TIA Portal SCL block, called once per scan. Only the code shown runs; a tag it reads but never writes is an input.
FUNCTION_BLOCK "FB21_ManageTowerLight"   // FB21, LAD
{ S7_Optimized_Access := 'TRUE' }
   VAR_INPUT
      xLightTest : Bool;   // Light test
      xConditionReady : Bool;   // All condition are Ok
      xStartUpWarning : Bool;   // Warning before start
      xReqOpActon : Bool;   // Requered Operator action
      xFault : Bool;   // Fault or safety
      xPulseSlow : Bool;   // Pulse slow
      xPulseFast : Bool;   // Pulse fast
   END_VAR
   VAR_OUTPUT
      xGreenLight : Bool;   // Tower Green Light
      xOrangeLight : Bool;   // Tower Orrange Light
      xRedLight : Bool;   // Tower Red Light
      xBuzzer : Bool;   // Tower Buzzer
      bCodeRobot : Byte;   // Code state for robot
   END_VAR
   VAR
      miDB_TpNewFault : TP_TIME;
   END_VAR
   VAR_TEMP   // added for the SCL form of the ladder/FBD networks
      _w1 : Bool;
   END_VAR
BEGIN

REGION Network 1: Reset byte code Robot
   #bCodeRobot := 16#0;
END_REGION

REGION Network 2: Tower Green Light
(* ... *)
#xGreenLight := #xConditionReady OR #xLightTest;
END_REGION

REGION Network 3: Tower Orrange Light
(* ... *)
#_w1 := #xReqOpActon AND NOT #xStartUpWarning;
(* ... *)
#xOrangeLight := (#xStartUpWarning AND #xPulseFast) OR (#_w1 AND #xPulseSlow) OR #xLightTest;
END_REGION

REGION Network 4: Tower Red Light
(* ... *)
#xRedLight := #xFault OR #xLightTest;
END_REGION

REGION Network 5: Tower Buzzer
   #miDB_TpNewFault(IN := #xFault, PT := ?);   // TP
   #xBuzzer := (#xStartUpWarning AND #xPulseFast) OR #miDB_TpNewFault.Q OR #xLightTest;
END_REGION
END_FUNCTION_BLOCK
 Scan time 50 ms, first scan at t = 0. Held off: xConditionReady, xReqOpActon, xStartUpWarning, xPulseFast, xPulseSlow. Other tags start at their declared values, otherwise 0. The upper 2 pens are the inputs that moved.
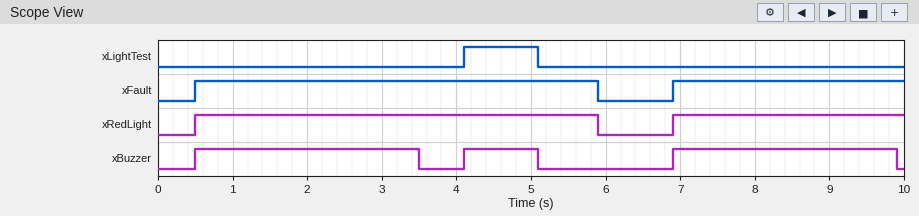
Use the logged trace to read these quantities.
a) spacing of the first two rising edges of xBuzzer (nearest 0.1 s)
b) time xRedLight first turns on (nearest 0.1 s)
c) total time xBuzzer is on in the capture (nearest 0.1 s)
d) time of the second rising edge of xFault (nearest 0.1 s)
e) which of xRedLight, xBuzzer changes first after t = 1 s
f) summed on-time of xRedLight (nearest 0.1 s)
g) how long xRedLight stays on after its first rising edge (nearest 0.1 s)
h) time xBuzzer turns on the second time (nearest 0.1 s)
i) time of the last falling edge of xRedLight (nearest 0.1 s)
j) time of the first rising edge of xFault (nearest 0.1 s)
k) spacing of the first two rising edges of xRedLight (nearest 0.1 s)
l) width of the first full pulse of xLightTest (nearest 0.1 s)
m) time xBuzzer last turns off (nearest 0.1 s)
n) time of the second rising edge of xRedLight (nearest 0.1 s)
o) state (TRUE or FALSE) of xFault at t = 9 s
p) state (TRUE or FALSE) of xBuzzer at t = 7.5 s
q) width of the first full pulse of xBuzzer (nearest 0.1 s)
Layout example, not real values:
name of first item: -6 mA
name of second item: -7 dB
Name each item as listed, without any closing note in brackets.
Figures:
spacing of the first two rising edges of xBuzzer: 3.6 s
time xRedLight first turns on: 0.5 s
total time xBuzzer is on in the capture: 7.0 s
time of the second rising edge of xFault: 6.9 s
which of xRedLight, xBuzzer changes first after t = 1 s: xBuzzer
summed on-time of xRedLight: 8.5 s
how long xRedLight stays on after its first rising edge: 5.4 s
time xBuzzer turns on the second time: 4.1 s
time of the last falling edge of xRedLight: 5.9 s
time of the first rising edge of xFault: 0.5 s
spacing of the first two rising edges of xRedLight: 6.4 s
width of the first full pulse of xLightTest: 1.0 s
time xBuzzer last turns off: 9.9 s
time of the second rising edge of xRedLight: 6.9 s
state (TRUE or FALSE) of xFault at t = 9 s: TRUE
state (TRUE or FALSE) of xBuzzer at t = 7.5 s: TRUE
width of the first full pulse of xBuzzer: 3.0 s
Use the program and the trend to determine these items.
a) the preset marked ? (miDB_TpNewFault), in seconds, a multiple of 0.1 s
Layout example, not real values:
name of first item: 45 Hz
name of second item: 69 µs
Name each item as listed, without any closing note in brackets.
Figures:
the preset marked ? (miDB_TpNewFault), in seconds, a multiple of 0.1 s: 3.0 s
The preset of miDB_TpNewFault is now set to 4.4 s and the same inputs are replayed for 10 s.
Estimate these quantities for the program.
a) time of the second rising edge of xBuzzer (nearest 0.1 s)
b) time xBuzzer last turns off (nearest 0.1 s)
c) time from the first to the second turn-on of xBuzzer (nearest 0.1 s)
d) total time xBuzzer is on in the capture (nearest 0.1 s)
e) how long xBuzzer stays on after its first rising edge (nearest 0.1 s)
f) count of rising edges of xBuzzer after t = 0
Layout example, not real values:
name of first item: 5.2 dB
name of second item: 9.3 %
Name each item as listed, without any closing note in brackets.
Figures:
time of the second rising edge of xBuzzer: 6.9 s
time xBuzzer last turns off: 5.1 s
time from the first to the second turn-on of xBuzzer: 6.4 s
total time xBuzzer is on in the capture: 7.7 s
how long xBuzzer stays on after its first rising edge: 4.6 s
count of rising edges of xBuzzer after t = 0: 2
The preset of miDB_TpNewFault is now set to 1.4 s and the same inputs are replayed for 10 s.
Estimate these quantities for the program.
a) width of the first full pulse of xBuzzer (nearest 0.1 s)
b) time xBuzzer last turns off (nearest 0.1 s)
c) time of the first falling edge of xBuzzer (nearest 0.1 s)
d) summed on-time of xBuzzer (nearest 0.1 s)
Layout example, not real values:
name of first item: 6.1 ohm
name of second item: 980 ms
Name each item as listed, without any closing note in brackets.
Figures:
width of the first full pulse of xBuzzer: 1.4 s
time xBuzzer last turns off: 8.3 s
time of the first falling edge of xBuzzer: 1.9 s
summed on-time of xBuzzer: 3.8 s
